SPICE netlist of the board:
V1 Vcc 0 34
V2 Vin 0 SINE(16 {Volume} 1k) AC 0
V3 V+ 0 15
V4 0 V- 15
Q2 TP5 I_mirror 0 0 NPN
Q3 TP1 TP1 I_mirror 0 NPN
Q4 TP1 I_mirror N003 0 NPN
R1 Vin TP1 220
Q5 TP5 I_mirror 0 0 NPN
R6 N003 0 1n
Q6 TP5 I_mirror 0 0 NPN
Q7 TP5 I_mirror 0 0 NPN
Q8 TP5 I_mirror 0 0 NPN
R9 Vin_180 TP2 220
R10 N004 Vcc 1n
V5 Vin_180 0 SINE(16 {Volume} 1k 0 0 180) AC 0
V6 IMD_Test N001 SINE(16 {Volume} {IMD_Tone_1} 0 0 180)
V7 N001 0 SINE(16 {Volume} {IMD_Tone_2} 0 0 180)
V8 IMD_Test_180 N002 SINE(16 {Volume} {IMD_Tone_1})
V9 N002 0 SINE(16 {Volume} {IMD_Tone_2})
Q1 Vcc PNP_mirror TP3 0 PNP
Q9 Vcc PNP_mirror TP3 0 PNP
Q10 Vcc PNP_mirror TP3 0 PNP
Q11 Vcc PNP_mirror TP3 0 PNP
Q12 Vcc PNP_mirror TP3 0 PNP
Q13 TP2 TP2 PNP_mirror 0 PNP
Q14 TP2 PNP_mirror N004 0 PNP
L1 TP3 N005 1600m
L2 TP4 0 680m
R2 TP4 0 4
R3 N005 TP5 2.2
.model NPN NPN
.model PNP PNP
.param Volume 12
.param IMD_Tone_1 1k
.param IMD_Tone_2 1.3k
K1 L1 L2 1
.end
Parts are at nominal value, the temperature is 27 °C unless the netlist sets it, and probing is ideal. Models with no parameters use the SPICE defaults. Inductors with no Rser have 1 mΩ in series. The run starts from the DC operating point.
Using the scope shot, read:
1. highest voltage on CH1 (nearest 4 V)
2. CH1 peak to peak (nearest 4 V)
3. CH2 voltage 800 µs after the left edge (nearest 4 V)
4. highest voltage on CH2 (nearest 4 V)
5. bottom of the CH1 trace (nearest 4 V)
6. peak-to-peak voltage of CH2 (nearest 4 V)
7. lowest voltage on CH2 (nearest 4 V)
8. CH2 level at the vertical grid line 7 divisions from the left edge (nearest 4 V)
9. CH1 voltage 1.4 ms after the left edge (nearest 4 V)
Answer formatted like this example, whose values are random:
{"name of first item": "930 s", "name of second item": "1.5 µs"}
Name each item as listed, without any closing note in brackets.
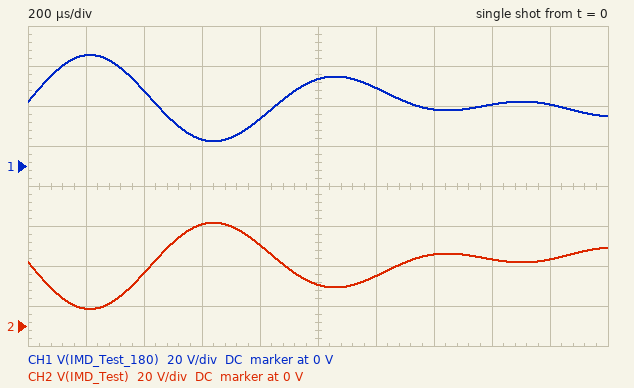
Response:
{"highest voltage on CH1": "56 V", "CH1 peak to peak": "44 V", "CH2 voltage 800 µs after the left edge": "40 V", "highest voltage on CH2": "52 V", "bottom of the CH1 trace": "12 V", "peak-to-peak voltage of CH2": "44 V", "lowest voltage on CH2": "8 V", "CH2 level at the vertical grid line 7 divisions from the left edge": "36 V", "CH1 voltage 1.4 ms after the left edge": "28 V"}
